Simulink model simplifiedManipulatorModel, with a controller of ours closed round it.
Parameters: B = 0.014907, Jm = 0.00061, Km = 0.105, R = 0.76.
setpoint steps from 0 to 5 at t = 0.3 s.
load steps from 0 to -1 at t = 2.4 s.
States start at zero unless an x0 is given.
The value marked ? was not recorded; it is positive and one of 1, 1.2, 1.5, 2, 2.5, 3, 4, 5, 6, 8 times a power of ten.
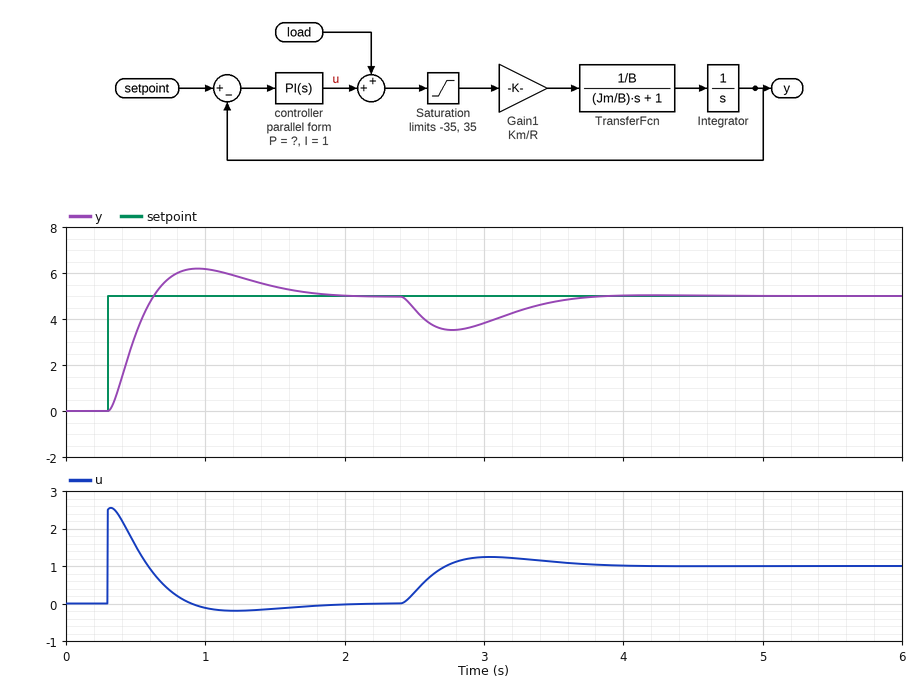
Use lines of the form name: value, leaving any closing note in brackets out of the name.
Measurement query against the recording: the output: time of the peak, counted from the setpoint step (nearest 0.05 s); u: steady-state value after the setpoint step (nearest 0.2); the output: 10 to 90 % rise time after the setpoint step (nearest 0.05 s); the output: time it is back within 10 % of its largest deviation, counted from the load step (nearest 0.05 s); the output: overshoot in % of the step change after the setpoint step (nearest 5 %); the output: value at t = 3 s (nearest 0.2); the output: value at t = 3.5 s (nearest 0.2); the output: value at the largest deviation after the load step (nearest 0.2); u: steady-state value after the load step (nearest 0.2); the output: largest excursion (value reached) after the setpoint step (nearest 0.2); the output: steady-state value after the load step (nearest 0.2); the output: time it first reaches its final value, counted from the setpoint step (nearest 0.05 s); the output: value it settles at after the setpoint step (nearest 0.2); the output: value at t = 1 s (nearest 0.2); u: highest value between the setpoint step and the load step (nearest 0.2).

the output: time of the peak, counted from the setpoint step: 0.65 s
u: steady-state value after the setpoint step: 0.0
the output: 10 to 90 % rise time after the setpoint step: 0.25 s
the output: time it is back within 10 % of its largest deviation, counted from the load step: 1.20 s
the output: overshoot in % of the step change after the setpoint step: 25 %
the output: value at t = 3 s: 3.8
the output: value at t = 3.5 s: 4.8
the output: value at the largest deviation after the load step: 3.6
u: steady-state value after the load step: 1.0
the output: largest excursion (value reached) after the setpoint step: 6.2
the output: steady-state value after the load step: 5.0
the output: time it first reaches its final value, counted from the setpoint step: 0.35 s
the output: value it settles at after the setpoint step: 5.0
the output: value at t = 1 s: 6.2
u: highest value between the setpoint step and the load step: 2.6
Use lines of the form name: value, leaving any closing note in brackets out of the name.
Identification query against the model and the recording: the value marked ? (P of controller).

the value marked ?: 0.5
